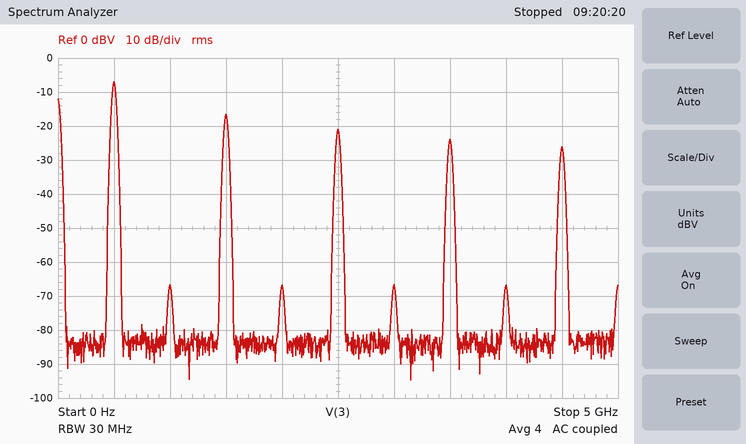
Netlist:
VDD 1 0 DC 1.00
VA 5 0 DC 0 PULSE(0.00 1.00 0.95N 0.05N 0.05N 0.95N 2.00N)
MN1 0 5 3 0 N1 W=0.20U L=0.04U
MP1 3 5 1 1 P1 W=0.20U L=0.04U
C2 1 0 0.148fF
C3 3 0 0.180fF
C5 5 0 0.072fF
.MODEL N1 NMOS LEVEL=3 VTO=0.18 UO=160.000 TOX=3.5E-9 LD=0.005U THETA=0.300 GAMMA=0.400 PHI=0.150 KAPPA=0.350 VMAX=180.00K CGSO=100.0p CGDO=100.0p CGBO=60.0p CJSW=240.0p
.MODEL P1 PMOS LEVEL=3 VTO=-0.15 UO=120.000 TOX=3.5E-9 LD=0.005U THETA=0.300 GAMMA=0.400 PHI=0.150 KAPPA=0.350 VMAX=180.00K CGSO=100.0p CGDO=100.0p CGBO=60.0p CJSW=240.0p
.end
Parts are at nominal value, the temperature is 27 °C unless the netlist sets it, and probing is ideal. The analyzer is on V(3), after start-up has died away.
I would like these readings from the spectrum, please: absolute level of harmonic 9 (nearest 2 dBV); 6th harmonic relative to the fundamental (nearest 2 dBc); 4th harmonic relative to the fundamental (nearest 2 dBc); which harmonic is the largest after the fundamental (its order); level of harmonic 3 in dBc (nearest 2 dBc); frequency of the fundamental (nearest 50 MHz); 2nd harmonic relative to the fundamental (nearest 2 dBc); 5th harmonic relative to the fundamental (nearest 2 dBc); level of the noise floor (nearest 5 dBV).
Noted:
-26 dBV
-60 dBc
-60 dBc
3
-10 dBc
500 MHz
-60 dBc
-14 dBc
-85 dBV
